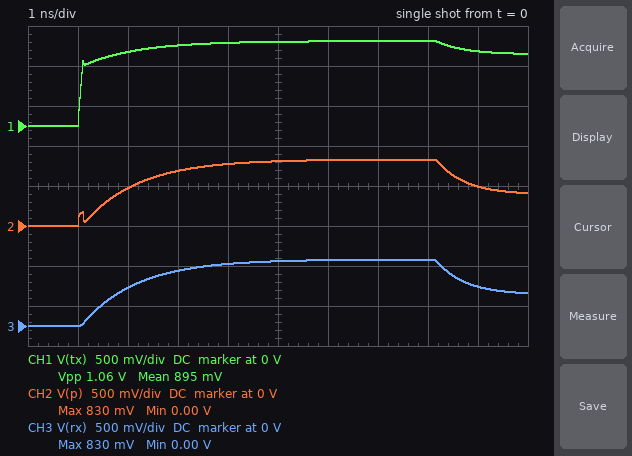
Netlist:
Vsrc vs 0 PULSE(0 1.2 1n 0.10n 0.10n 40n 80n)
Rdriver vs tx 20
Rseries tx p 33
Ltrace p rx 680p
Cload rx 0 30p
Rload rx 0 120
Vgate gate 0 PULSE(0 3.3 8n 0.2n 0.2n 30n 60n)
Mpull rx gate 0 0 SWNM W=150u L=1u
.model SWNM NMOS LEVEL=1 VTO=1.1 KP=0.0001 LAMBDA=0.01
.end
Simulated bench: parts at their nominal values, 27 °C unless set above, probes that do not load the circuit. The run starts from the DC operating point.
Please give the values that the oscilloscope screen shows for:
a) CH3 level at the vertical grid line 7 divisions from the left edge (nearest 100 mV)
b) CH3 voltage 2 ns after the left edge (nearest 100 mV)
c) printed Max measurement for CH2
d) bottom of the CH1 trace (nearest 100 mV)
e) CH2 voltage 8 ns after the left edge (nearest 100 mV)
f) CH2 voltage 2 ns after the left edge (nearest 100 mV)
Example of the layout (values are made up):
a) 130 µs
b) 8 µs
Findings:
a) 800 mV
b) 500 mV
c) 830 mV
d) 0 V
e) 800 mV
f) 500 mV
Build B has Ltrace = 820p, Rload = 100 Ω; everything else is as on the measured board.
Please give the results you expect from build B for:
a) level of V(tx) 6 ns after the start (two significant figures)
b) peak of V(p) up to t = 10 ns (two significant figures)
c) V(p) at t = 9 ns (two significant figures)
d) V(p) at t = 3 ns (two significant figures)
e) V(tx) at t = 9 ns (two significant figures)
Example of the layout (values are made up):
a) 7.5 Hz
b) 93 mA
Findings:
a) 1.0 V
b) 780 mV
c) 470 mV
d) 660 mV
e) 920 mV
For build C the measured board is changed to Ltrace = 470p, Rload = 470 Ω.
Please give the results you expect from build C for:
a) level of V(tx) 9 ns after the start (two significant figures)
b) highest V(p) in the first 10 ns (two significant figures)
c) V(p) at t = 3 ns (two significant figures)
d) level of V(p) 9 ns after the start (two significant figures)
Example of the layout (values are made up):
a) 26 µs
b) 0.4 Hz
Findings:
a) 980 mV
b) 1.1 V
c) 800 mV
d) 620 mV
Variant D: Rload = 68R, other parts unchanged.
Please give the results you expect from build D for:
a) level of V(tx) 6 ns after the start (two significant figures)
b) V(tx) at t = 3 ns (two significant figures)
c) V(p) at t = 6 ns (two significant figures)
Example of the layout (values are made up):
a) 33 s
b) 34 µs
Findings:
a) 1.0 V
b) 970 mV
c) 670 mV
